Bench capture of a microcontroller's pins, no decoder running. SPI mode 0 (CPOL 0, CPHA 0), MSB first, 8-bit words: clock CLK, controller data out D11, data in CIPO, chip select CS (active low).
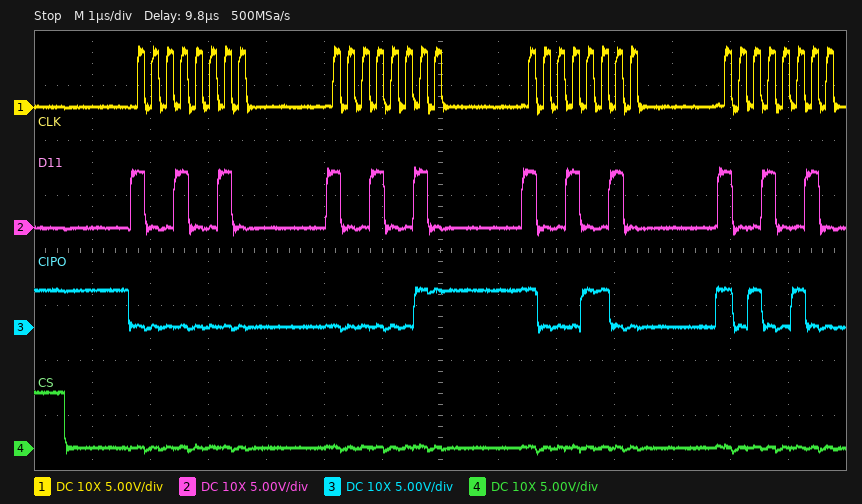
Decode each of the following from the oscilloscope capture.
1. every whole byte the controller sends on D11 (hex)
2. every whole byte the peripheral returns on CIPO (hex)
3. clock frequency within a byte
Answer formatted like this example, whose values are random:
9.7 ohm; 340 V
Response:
92 92 92 92; 00 03 8C A4; 4 MHz
